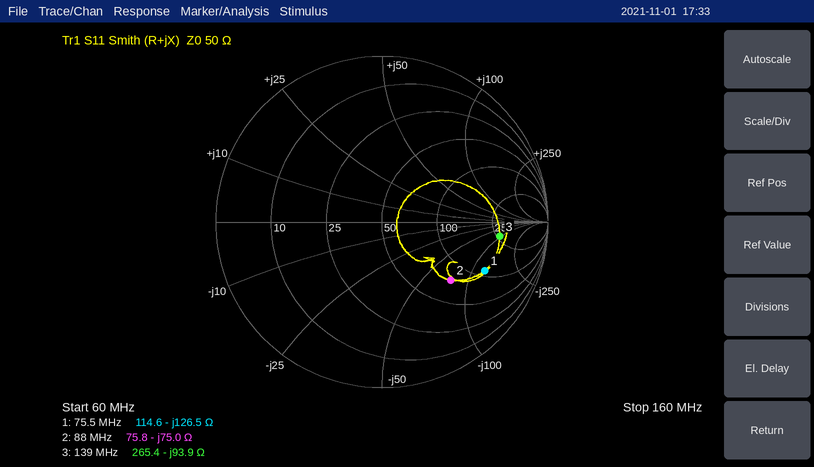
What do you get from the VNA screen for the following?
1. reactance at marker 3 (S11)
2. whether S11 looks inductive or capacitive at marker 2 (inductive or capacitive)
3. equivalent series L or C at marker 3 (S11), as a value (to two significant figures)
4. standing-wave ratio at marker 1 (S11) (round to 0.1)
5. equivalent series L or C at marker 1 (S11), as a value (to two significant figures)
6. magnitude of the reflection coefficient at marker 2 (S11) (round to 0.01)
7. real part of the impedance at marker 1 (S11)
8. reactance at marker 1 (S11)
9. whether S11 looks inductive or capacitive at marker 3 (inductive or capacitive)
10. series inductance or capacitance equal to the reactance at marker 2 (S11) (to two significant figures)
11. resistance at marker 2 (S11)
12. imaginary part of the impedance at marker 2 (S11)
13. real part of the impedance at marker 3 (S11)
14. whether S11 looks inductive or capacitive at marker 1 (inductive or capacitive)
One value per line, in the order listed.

-93.9 Ω
capacitive
12 pF
5.3
17 pF
0.54
114.6 Ω
-126.5 Ω
capacitive
24 pF
75.8 Ω
-75.0 Ω
265.4 Ω
capacitive
